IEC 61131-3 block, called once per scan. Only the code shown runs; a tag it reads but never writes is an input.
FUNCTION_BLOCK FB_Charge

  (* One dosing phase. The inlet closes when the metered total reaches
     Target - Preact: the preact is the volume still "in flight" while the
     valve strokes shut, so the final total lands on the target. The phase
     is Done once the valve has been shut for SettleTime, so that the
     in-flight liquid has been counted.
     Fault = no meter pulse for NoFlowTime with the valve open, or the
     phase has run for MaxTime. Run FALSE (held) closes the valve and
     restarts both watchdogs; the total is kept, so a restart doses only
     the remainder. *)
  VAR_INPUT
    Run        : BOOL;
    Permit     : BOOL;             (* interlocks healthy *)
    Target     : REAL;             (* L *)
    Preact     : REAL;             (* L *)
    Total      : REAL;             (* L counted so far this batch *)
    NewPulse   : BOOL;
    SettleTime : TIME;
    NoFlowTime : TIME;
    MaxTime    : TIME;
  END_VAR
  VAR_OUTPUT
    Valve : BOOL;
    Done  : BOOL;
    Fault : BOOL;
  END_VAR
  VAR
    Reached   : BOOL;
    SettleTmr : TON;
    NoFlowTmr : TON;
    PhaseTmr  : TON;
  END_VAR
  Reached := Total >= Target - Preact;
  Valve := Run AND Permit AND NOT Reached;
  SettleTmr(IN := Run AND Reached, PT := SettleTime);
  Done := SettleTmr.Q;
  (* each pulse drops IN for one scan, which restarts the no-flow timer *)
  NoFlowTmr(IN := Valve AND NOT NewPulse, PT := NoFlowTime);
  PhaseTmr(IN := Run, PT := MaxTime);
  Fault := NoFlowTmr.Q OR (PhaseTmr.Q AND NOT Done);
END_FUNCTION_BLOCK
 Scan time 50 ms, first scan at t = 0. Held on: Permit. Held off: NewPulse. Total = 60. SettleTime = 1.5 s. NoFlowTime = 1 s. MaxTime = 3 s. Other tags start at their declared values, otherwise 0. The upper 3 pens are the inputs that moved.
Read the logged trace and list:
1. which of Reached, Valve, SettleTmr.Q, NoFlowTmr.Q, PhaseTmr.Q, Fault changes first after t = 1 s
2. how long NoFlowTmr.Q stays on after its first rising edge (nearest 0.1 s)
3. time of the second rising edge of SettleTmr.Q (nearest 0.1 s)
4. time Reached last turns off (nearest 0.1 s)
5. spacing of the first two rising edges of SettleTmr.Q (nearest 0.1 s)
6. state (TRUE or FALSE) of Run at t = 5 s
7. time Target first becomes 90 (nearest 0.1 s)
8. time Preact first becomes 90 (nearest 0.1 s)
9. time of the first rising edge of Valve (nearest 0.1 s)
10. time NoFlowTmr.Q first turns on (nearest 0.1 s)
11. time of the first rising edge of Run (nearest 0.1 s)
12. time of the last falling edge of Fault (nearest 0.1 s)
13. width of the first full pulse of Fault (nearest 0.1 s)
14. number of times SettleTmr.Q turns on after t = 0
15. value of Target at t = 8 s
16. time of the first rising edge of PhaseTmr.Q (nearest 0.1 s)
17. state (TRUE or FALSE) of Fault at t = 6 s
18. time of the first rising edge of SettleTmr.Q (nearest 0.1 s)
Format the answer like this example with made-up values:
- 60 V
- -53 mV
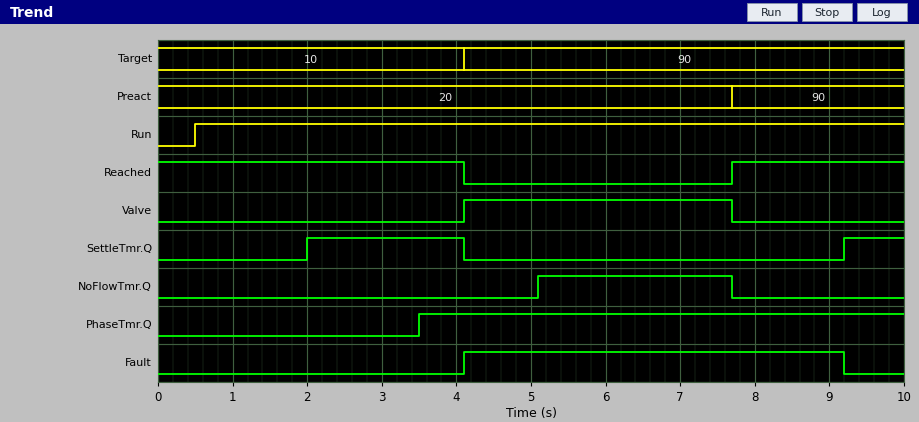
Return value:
- SettleTmr.Q
- 2.6 s
- 9.2 s
- 4.1 s
- 7.2 s
- TRUE
- 4.1 s
- 7.7 s
- 4.1 s
- 5.1 s
- 0.5 s
- 9.2 s
- 5.1 s
- 2
- 90
- 3.5 s
- TRUE
- 2.0 s
